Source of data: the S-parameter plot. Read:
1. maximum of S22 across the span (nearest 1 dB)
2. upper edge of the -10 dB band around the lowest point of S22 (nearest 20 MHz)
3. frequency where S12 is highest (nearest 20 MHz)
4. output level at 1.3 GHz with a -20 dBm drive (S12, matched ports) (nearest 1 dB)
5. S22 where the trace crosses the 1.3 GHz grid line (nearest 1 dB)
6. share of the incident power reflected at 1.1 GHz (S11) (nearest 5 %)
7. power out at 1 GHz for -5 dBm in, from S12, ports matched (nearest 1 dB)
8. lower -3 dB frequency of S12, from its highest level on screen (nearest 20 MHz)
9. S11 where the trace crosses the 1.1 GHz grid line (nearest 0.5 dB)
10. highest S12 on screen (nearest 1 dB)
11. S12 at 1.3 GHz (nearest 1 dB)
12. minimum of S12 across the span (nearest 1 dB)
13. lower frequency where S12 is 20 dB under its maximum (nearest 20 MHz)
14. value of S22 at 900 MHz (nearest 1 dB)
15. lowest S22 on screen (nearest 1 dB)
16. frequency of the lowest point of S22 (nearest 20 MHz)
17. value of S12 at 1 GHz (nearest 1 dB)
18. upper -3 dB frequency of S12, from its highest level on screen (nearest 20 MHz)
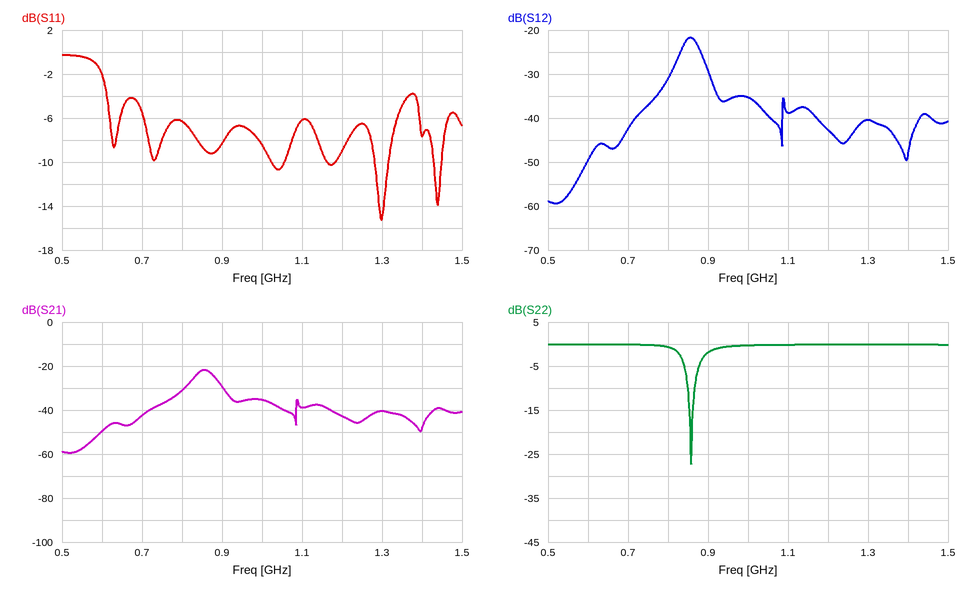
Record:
0 dB
860 MHz
860 MHz
-60 dBm
0 dB
25 %
-40 dBm
840 MHz
-6.0 dB
-22 dB
-40 dB
-59 dB
700 MHz
-2 dB
-27 dB
860 MHz
-35 dB
880 MHz
